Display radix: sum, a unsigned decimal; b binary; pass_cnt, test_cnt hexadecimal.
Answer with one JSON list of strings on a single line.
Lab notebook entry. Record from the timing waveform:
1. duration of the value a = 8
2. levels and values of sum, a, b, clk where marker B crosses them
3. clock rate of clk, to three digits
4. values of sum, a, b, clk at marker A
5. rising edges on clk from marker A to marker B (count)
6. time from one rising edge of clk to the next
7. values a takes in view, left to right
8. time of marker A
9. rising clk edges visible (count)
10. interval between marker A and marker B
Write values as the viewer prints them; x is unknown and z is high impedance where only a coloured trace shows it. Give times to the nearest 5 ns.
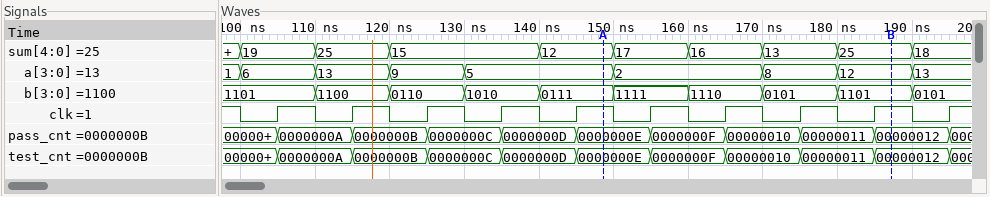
["10 ns", "sum=25, a=12, b=1101, clk=1", "100 MHz", "sum=12, a=5, b=0111, clk=1", "4", "10 ns", "1, 6, 13, 9, 5, 2, 8, 12, 13", "150 ns", "10", "40 ns"]
